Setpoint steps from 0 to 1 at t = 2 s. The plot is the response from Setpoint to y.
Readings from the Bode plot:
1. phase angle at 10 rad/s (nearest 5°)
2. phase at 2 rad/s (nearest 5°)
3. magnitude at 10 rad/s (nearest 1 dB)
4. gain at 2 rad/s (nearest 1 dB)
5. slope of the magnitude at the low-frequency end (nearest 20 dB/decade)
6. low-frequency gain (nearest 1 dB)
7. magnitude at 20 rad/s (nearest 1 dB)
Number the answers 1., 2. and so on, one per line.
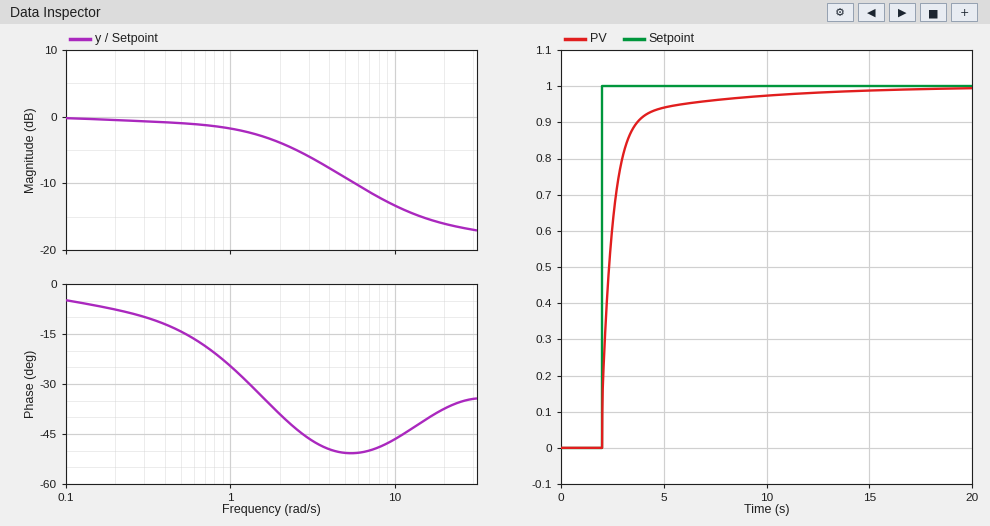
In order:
1. -45°
2. -40°
3. -13 dB
4. -4 dB
5. 0 dB/decade
6. 0 dB
7. -16 dB
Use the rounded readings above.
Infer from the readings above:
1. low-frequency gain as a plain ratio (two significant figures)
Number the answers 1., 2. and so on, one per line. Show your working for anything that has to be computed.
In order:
1. 10^(0 / 20) = 1.0
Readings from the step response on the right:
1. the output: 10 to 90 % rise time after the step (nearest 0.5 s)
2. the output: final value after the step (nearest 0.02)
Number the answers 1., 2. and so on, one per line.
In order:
1. 1.5 s
2. 1.00
